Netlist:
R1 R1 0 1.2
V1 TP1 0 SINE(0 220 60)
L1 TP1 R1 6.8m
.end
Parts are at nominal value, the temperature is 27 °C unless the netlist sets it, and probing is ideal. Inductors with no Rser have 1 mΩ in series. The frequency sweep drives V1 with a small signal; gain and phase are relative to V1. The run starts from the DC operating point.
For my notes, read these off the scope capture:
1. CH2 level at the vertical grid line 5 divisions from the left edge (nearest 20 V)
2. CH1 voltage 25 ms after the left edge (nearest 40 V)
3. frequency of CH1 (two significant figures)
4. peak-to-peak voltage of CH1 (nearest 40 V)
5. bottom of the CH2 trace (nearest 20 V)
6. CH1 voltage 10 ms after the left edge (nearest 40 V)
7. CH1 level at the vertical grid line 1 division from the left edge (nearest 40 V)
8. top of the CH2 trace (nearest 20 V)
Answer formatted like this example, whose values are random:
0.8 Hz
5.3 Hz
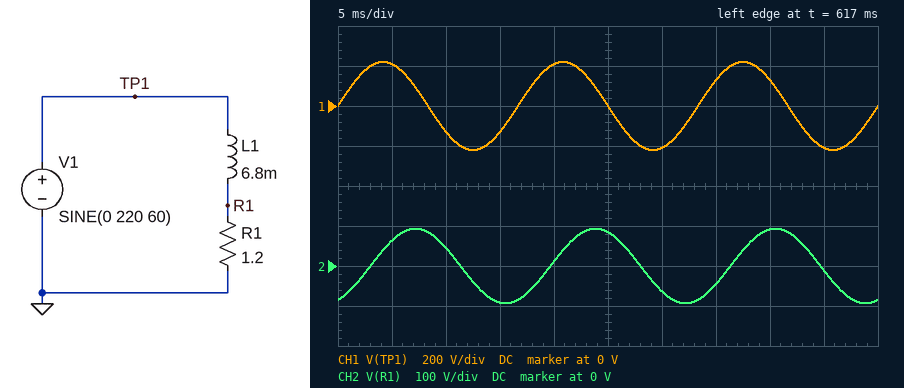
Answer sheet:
80 V
0 V
60 Hz
440 V
-100 V
-120 V
200 V
100 V
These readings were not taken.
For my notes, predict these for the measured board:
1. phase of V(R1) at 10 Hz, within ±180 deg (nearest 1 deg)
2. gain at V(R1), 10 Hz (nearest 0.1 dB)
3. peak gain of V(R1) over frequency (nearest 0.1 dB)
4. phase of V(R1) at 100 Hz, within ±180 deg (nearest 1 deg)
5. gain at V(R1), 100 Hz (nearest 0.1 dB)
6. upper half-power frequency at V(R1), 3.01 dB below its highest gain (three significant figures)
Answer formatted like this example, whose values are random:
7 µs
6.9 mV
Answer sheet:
-20 deg
-0.5 dB
0 dB
-74 deg
-11.4 dB
28.1 Hz
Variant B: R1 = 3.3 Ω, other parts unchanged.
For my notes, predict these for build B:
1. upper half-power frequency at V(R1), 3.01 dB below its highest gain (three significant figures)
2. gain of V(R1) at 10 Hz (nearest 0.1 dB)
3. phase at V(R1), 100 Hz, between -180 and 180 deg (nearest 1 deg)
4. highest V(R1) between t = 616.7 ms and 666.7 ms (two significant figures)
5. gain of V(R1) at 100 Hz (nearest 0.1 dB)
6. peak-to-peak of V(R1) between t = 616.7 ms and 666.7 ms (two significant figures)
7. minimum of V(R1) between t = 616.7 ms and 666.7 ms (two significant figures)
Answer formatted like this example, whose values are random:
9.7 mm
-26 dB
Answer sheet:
77.3 Hz
-0.1 dB
-52 deg
170 V
-4.3 dB
350 V
-170 V
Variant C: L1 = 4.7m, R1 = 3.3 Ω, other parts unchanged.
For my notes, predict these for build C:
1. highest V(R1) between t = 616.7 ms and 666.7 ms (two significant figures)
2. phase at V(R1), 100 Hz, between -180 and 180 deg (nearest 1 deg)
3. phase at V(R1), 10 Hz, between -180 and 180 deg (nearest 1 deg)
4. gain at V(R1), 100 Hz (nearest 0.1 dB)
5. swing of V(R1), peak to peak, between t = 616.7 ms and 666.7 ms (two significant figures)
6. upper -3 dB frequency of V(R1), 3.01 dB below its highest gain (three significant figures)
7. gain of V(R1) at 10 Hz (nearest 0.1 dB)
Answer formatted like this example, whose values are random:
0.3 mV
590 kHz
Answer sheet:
190 V
-42 deg
-5 deg
-2.6 dB
390 V
112 Hz
0 dB
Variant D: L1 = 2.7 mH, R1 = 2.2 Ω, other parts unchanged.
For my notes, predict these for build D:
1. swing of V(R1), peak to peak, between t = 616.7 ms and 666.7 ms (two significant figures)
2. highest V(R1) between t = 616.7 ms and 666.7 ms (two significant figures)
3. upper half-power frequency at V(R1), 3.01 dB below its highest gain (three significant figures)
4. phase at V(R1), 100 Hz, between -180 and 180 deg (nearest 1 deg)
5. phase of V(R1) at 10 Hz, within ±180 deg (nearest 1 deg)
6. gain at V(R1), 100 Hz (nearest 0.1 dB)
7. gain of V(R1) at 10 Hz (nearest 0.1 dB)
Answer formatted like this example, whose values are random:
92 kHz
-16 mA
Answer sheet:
400 V
200 V
130 Hz
-38 deg
-4 deg
-2.0 dB
0 dB
